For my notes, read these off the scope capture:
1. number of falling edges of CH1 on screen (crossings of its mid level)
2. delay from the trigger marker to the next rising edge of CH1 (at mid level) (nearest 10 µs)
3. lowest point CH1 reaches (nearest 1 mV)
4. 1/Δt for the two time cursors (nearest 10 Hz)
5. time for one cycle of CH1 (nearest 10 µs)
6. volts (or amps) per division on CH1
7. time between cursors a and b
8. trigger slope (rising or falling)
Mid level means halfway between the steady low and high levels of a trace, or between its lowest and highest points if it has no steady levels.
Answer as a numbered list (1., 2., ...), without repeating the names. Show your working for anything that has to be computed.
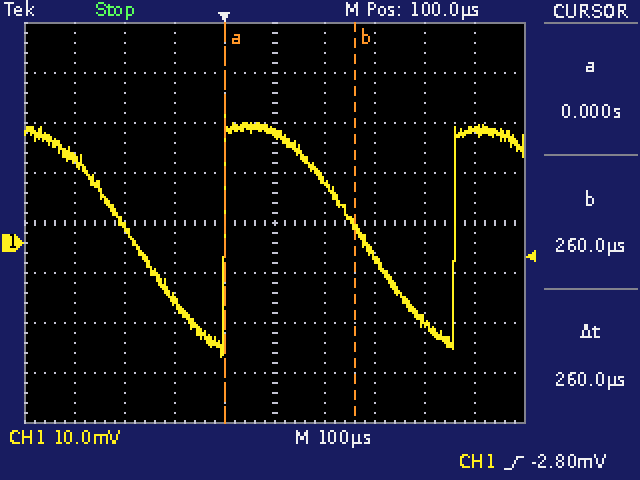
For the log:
1. 2
2. 460 µs
3. -23 mV
4. 1 / 260 µs ≈ 3.85 kHz
5. 460 µs
6. 10 mV
7. 260 µs
8. rising
